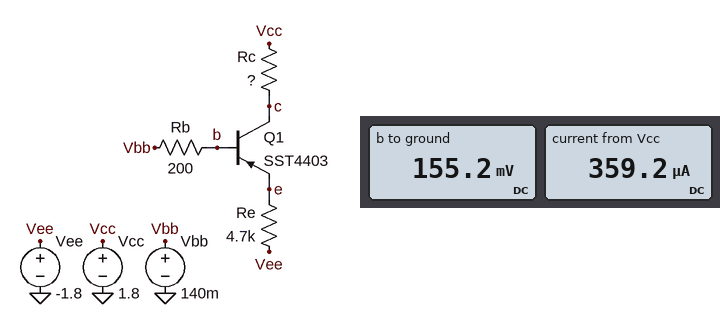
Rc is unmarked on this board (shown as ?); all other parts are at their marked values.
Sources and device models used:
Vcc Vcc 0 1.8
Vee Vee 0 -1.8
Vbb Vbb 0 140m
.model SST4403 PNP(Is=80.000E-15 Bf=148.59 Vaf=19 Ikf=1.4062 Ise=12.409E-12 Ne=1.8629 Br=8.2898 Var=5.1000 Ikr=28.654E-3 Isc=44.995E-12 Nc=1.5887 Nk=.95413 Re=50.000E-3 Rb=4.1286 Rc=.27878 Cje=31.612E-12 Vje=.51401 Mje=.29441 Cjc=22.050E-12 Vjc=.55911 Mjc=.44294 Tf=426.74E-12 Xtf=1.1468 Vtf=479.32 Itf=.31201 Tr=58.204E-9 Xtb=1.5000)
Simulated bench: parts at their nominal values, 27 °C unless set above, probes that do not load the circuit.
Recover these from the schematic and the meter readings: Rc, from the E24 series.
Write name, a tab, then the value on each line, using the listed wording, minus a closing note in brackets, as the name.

Rc, from the E24 series	3 kΩ
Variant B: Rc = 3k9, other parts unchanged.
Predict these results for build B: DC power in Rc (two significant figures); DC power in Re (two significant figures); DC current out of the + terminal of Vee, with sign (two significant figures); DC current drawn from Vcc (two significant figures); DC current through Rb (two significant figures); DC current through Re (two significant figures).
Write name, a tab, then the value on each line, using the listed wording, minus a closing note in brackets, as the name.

DC power in Rc	300 µW
DC power in Re	230 µW
DC current out of the + terminal of Vee, with sign	-220 µA
DC current drawn from Vcc	280 µA
DC current through Rb	60 µA
DC current through Re	220 µA
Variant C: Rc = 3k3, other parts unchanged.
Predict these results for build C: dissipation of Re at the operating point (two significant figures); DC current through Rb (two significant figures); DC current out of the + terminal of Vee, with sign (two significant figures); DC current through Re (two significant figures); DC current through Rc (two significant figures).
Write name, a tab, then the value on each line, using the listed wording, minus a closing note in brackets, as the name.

dissipation of Re at the operating point	310 µW
DC current through Rb	69 µA
DC current out of the + terminal of Vee, with sign	-260 µA
DC current through Re	260 µA
DC current through Rc	330 µA
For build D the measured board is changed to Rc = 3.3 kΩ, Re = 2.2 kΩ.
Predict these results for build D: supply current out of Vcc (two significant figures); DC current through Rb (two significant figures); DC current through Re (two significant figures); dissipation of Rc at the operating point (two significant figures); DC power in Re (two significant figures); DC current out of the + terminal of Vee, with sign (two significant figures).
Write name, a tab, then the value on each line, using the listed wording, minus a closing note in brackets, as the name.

supply current out of Vcc	330 µA
DC current through Rb	65 µA
DC current through Re	260 µA
dissipation of Rc at the operating point	360 µW
DC power in Re	150 µW
DC current out of the + terminal of Vee, with sign	-260 µA
